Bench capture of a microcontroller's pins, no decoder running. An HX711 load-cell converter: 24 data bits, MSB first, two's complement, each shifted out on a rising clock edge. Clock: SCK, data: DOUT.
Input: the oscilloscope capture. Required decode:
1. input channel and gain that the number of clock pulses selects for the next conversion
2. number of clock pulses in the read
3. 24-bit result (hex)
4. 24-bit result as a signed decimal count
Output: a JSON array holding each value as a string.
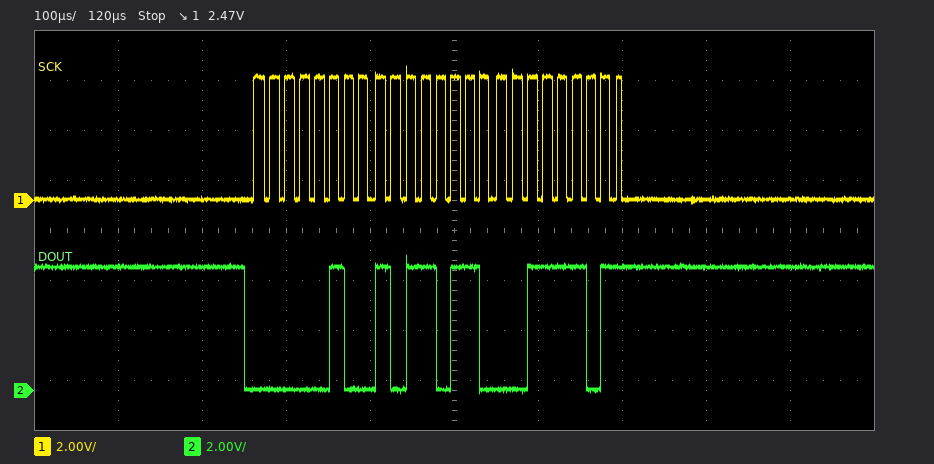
["channel A, gain 128", "25", "0x04B63D", "308797"]
